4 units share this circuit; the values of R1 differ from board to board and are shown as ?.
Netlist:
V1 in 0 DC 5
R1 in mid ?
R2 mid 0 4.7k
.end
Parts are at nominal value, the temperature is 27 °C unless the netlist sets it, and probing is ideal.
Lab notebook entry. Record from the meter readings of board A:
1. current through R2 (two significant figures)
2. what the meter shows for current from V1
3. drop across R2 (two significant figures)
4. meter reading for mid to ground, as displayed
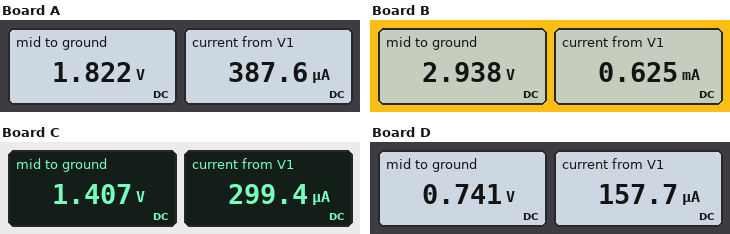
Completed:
390 µA
387.6 µA
1.8 V
1.822 V
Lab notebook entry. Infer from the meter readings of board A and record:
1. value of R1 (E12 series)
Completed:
8.2 kΩ
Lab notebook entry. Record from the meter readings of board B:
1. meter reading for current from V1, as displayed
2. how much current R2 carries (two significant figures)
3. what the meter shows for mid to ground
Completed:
0.625 mA
630 µA
2.938 V
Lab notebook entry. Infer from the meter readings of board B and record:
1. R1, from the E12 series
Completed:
3.3 kΩ
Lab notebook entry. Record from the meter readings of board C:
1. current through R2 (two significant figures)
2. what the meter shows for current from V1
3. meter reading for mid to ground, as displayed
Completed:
300 µA
299.4 µA
1.407 V
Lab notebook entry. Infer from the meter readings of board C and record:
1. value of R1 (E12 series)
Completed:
12 kΩ
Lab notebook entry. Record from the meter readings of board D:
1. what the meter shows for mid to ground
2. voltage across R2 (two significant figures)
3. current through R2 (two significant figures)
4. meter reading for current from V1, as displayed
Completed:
0.741 V
740 mV
160 µA
157.7 µA
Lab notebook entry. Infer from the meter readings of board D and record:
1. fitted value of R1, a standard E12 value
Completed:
27 kΩ
